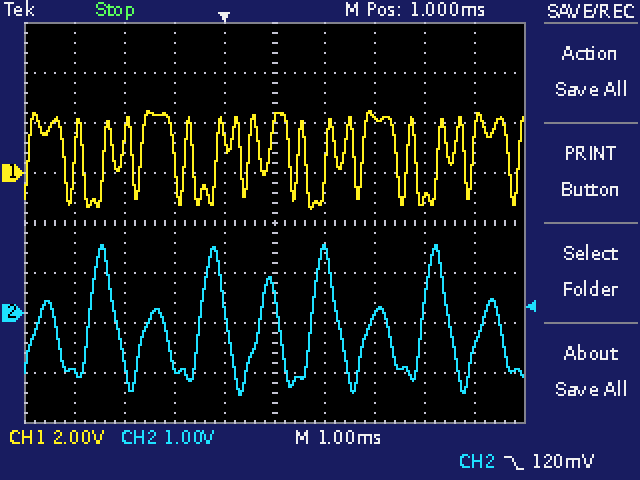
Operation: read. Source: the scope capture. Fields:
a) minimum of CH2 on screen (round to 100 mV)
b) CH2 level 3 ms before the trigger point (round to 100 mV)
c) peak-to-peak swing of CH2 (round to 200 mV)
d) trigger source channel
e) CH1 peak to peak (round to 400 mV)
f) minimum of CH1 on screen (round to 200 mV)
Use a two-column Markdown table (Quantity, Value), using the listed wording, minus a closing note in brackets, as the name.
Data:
| Quantity | Value |
|---|---|
| minimum of CH2 on screen | -1.6 V |
| CH2 level 3 ms before the trigger point | -1.2 V |
| peak-to-peak swing of CH2 | 3.0 V |
| trigger source channel | CH2 |
| CH1 peak to peak | 4.0 V |
| minimum of CH1 on screen | -1.4 V |
